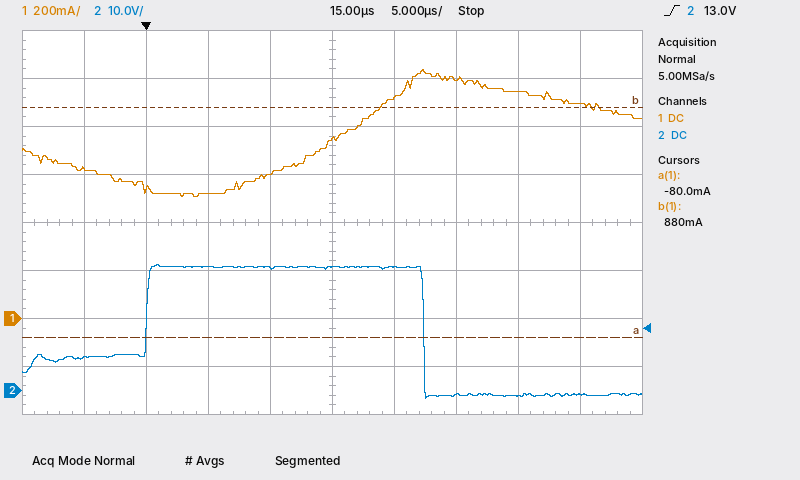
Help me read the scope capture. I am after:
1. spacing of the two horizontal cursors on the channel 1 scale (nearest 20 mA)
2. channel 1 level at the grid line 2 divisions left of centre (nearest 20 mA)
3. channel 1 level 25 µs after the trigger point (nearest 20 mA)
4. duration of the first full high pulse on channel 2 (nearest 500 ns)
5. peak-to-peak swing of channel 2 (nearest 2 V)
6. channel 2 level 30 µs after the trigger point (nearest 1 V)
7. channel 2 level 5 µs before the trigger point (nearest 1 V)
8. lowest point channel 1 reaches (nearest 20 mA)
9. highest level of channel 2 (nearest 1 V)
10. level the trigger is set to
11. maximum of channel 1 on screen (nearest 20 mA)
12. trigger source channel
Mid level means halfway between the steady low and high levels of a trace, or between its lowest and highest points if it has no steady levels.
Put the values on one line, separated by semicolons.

960 mA; 520 mA; 1.00 A; 22.5 µs; 28 V; -1 V; 7 V; 500 mA; 26 V; 13.0 V; 1.04 A; channel 2
